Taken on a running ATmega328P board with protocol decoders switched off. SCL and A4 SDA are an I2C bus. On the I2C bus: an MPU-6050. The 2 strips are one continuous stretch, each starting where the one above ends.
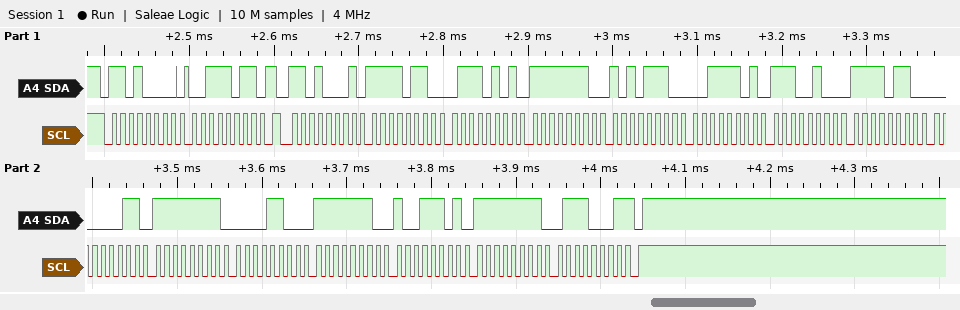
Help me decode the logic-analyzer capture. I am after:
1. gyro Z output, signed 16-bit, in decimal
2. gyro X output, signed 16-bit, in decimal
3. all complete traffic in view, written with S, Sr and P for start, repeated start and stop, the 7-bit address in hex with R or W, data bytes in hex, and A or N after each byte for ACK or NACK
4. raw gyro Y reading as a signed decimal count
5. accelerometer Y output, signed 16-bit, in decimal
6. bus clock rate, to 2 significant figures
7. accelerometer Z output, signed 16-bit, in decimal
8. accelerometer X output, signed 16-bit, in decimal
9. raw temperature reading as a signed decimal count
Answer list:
-143
-244
S 68W A 3B A Sr 68R A F6 A 75 A FE A AE A 3D A E4 A F6 A 03 A FF A 0C A FE A 9D A FF A 71 N P
-355
-338
100 kHz
15844
-2443
-2557
